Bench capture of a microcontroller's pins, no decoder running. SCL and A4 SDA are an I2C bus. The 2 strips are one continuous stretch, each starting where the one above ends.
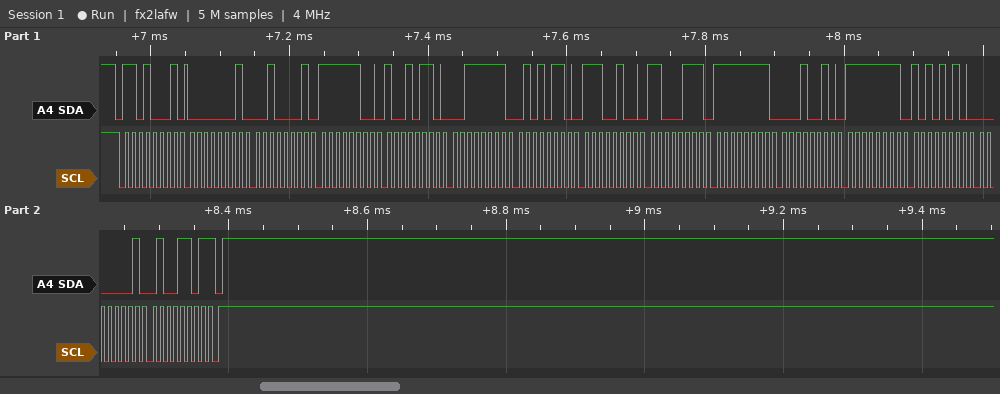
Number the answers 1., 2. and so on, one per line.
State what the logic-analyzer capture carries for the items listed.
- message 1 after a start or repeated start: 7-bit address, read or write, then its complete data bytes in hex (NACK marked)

1. 0x68 read: 01 21 FC 96 3F 56 E4 C7 FF 12 FF AA 01 4D NACK
